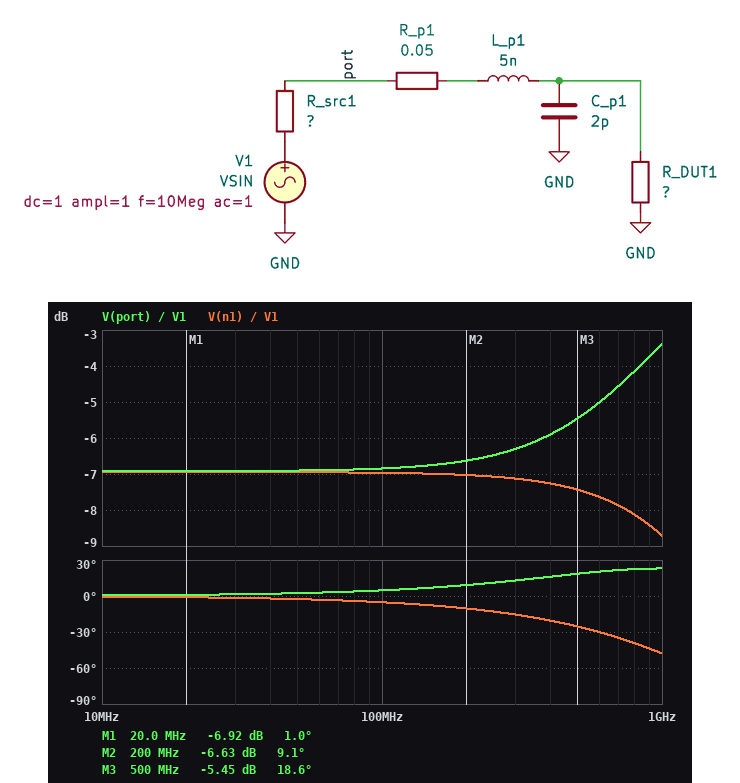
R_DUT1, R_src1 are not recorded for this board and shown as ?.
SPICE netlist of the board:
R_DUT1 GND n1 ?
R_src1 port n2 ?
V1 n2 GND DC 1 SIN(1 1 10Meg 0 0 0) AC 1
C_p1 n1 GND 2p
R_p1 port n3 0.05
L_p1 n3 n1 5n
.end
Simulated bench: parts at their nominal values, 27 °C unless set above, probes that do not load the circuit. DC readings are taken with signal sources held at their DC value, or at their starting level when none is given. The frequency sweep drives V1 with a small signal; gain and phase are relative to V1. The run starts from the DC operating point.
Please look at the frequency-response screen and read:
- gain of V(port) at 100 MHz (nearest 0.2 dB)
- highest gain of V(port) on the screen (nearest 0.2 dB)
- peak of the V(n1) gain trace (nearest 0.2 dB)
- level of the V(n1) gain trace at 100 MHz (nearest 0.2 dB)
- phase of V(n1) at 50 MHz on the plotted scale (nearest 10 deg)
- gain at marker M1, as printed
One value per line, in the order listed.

-6.8 dB
-3.4 dB
-7.0 dB
-7.0 dB
0 deg
-6.92 dB
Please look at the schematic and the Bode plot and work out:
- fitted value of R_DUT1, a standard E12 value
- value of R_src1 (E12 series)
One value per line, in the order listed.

18 Ω
22 Ω
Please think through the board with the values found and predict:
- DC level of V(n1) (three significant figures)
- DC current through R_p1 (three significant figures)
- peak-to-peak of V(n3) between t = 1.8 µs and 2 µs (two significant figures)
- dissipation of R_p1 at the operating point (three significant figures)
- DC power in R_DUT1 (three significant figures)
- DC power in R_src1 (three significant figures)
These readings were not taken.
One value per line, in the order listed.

449 mV
25.0 mA
900 mV
31.2 µW
11.2 mW
13.7 mW
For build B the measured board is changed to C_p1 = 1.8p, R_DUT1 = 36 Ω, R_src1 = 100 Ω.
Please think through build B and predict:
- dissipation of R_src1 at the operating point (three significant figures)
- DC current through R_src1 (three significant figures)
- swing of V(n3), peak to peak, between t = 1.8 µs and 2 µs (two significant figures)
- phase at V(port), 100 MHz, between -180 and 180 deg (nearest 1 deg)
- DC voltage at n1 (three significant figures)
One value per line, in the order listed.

5.40 mW
7.35 mA
530 mV
2 deg
265 mV
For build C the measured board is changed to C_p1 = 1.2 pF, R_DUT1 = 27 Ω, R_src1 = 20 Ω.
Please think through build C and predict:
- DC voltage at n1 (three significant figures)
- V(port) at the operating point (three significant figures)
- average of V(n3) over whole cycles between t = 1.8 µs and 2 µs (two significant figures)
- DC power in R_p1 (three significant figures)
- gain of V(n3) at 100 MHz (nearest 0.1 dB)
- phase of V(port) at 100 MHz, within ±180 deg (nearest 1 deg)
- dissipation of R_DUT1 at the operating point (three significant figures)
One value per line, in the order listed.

574 mV
575 mV
570 mV
22.6 µW
-4.8 dB
2 deg
12.2 mW
